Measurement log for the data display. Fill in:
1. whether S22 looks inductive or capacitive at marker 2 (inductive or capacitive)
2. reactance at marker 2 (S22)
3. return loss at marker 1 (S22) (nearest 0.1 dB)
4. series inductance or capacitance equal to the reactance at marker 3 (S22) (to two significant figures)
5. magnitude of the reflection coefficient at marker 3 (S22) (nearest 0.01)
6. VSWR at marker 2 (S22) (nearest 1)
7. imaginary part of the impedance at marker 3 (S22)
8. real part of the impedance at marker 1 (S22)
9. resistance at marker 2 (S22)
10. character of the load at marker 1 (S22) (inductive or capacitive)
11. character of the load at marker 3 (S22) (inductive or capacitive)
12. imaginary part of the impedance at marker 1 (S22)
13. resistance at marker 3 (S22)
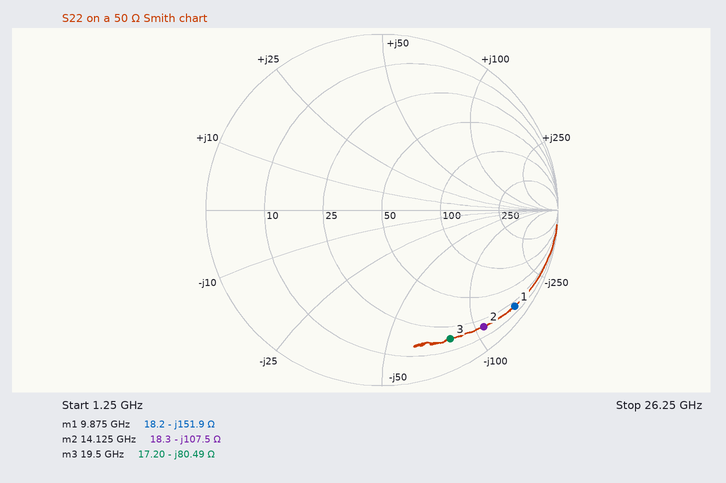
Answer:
capacitive
-107.5 Ω
0.6 dB
100 fF
0.83
16
-80.49 Ω
18.2 Ω
18.3 Ω
capacitive
capacitive
-151.9 Ω
17.20 Ω
